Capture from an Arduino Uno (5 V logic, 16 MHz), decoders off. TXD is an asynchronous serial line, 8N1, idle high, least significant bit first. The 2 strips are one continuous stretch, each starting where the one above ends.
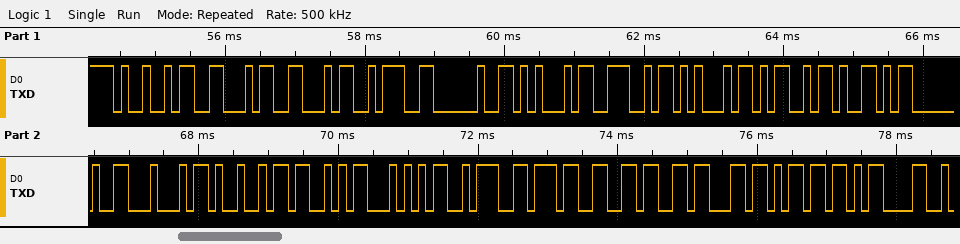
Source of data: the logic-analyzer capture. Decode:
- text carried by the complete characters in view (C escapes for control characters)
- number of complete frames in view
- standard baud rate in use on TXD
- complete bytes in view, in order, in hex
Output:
"IFF: ENEMY DIST:76cm\r"
21
9600 baud
49 46 46 3A 20 45 4E 45 4D 59 20 44 49 53 54 3A 37 36 63 6D 0D
